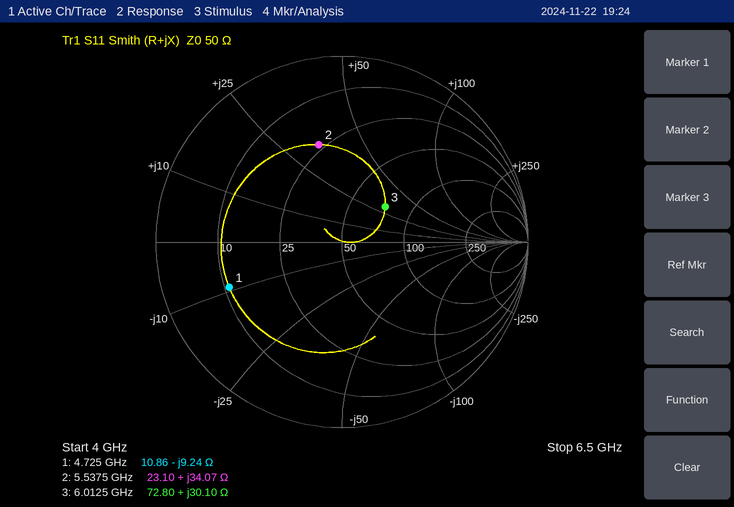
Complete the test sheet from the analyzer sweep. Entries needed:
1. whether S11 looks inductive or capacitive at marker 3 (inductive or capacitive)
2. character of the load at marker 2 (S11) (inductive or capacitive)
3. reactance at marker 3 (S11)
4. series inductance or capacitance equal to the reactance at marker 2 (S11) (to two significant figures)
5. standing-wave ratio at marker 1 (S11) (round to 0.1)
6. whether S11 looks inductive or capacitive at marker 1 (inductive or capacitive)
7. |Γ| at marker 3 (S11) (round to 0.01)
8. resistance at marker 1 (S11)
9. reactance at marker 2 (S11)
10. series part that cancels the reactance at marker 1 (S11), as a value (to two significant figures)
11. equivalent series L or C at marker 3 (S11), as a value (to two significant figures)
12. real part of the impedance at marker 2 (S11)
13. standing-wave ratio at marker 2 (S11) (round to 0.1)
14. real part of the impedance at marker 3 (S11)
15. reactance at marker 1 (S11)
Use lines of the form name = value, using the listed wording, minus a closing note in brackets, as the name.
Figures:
whether S11 looks inductive or capacitive at marker 3 = inductive
character of the load at marker 2 (S11) = inductive
reactance at marker 3 = +30.10 Ω
series inductance or capacitance equal to the reactance at marker 2 (S11) = 980 pH
standing-wave ratio at marker 1 (S11) = 4.8
whether S11 looks inductive or capacitive at marker 1 = capacitive
|Γ| at marker 3 (S11) = 0.30
resistance at marker 1 = 10.86 Ω
reactance at marker 2 = +34.07 Ω
series part that cancels the reactance at marker 1 (S11), as a value = 310 pH
equivalent series L or C at marker 3 (S11), as a value = 800 pH
real part of the impedance at marker 2 = 23.10 Ω
standing-wave ratio at marker 2 (S11) = 3.3
real part of the impedance at marker 3 = 72.80 Ω
reactance at marker 1 = -9.24 Ω
